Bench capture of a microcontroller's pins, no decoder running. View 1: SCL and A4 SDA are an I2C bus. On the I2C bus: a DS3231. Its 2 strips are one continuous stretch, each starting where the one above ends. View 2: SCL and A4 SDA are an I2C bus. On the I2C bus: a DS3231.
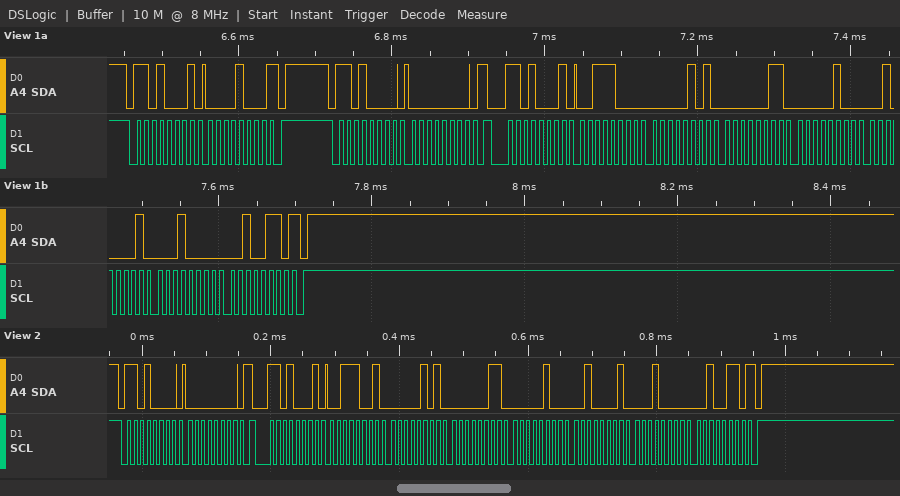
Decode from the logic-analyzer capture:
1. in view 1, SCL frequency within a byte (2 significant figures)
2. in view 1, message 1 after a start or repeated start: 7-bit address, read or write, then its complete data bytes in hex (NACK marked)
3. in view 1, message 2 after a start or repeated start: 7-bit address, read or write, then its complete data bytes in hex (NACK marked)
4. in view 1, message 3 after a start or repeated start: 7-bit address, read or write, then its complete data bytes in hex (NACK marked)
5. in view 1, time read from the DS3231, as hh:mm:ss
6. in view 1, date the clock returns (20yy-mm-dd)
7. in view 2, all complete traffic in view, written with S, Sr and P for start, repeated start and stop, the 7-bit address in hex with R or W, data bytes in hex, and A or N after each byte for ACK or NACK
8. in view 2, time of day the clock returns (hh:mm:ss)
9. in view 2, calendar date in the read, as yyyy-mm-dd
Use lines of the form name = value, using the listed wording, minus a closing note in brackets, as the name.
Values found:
in view 1, SCL frequency within a byte = 100 kHz
in view 1, message 1 after a start or repeated start: 7-bit address, read or write, then its complete data bytes in hex = 0x68 read: 08 NACK
in view 1, message 2 after a start or repeated start: 7-bit address, read or write, then its complete data bytes in hex = 0x68 write: 00
in view 1, message 3 after a start or repeated start: 7-bit address, read or write, then its complete data bytes in hex = 0x68 read: 38 05 03 04 21 10 26 NACK
in view 1, time read from the DS3231, as hh:mm:ss = 03:05:38
in view 1, date the clock returns = 2026-10-21
in view 2, all complete traffic in view, written with S, Sr and P for start, repeated start and stop, the 7-bit address in hex with R or W, data bytes in hex, and A or N after each byte for ACK or NACK = S 68W A 00 A Sr 68R A 39 A 05 A 03 A 04 A 21 A 10 A 26 N P
in view 2, time of day the clock returns = 03:05:39
in view 2, calendar date in the read, as yyyy-mm-dd = 2026-10-21
